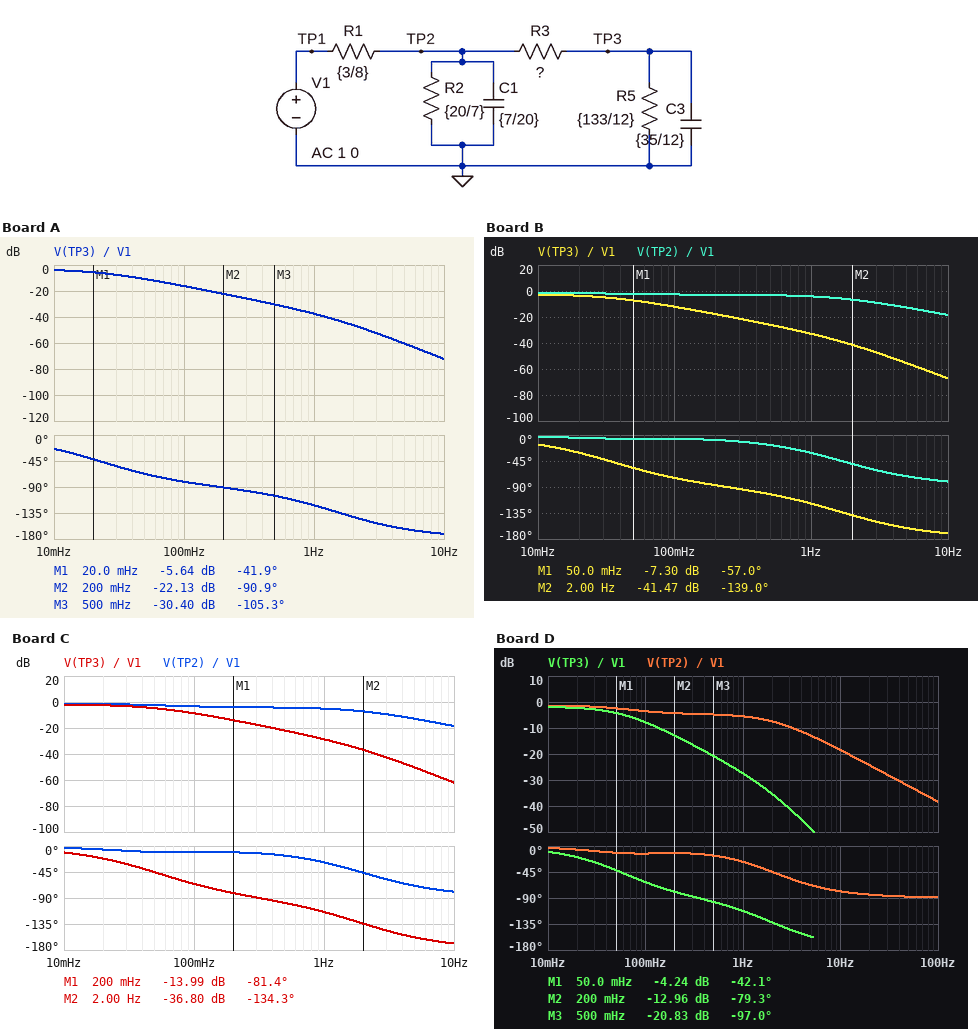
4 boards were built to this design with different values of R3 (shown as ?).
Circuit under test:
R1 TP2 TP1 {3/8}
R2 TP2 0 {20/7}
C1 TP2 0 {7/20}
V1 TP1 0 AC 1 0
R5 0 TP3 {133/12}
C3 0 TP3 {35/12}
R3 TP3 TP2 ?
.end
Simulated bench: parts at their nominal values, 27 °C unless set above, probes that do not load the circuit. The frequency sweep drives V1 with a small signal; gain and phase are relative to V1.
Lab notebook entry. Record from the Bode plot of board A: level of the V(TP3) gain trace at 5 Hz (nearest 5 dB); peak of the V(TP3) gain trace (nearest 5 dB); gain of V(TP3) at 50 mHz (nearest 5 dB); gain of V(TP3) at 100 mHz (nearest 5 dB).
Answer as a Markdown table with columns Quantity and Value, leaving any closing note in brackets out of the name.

| Quantity | Value |
|---|---|
| level of the V(TP3) gain trace at 5 Hz | -60 dB |
| peak of the V(TP3) gain trace | -5 dB |
| gain of V(TP3) at 50 mHz | -10 dB |
| gain of V(TP3) at 100 mHz | -15 dB |
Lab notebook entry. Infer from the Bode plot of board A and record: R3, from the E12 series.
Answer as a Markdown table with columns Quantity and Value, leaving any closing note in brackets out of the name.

| Quantity | Value |
|---|---|
| R3, from the E12 series | 2.7 Ω |
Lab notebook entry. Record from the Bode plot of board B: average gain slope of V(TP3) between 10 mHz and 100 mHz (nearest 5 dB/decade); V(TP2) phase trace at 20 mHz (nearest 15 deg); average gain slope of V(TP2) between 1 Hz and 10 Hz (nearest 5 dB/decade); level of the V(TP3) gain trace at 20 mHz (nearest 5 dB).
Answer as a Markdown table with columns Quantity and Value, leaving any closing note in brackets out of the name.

| Quantity | Value |
|---|---|
| average gain slope of V(TP3) between 10 mHz and 100 mHz | -10 dB/decade |
| V(TP2) phase trace at 20 mHz | 0 deg |
| average gain slope of V(TP2) between 1 Hz and 10 Hz | -15 dB/decade |
| level of the V(TP3) gain trace at 20 mHz | -5 dB |
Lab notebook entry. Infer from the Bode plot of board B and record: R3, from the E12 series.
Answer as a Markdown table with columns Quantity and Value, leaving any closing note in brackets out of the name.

| Quantity | Value |
|---|---|
| R3, from the E12 series | 1.5 Ω |
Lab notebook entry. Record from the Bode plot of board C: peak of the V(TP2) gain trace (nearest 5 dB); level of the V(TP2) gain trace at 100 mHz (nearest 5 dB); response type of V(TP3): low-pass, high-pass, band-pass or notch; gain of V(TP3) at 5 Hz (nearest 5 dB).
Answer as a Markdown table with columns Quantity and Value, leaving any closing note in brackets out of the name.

| Quantity | Value |
|---|---|
| peak of the V(TP2) gain trace | 0 dB |
| level of the V(TP2) gain trace at 100 mHz | -5 dB |
| response type of V(TP3): low-pass, high-pass, band-pass or notch | low-pass |
| gain of V(TP3) at 5 Hz | -50 dB |
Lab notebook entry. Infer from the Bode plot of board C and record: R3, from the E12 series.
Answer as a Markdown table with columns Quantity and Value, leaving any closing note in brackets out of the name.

| Quantity | Value |
|---|---|
| R3, from the E12 series | 0.82 Ω |
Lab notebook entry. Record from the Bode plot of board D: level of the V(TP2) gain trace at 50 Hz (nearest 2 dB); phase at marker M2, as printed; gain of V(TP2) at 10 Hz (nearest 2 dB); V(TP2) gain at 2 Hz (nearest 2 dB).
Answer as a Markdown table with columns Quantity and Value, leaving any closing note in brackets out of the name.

| Quantity | Value |
|---|---|
| level of the V(TP2) gain trace at 50 Hz | -32 dB |
| phase at marker M2, as printed | -79.3 deg |
| gain of V(TP2) at 10 Hz | -18 dB |
| V(TP2) gain at 2 Hz | -8 dB |
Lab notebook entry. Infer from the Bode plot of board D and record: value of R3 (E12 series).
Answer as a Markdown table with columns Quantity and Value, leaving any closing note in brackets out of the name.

| Quantity | Value |
|---|---|
| value of R3 | 0.68 Ω |
